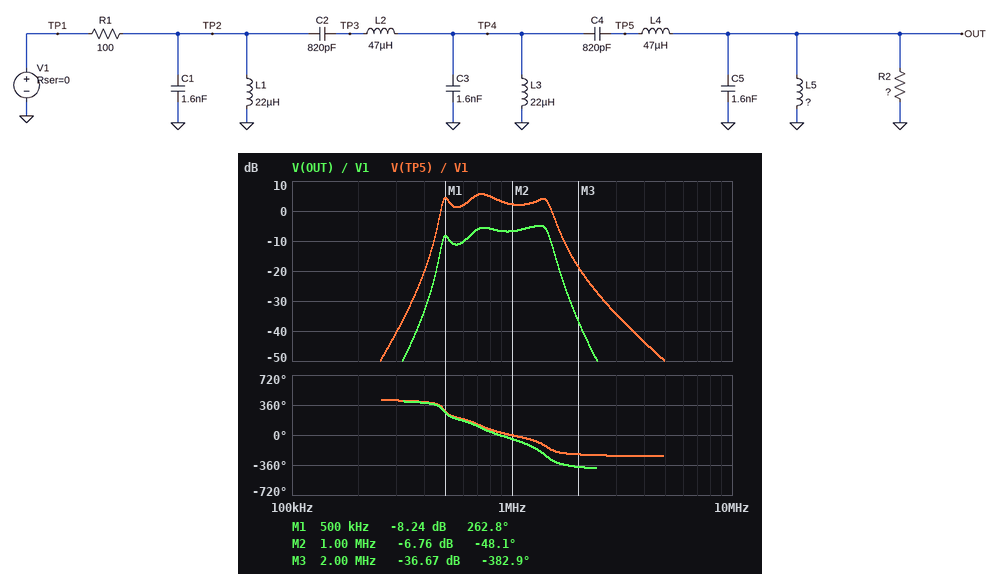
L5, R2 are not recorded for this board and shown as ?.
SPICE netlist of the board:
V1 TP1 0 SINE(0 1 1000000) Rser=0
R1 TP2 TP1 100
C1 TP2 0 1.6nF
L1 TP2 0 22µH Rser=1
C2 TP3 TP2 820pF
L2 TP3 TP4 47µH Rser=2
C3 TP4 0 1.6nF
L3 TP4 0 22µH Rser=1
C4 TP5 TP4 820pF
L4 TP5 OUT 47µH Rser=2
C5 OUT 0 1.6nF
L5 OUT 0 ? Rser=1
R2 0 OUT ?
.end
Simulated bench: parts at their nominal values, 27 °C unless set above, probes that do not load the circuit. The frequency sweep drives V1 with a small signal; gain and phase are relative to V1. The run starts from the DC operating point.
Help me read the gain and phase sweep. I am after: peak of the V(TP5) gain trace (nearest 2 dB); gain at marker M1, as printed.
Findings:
6 dB
-8.24 dB
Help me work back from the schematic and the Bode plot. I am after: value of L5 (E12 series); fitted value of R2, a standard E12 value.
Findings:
12 µH
150 Ω
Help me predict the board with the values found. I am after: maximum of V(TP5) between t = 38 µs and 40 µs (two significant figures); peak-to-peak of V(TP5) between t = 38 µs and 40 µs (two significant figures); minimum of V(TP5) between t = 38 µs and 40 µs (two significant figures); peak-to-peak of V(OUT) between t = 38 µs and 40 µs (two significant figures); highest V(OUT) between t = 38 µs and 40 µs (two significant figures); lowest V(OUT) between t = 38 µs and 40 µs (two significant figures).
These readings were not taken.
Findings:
1.3 V
2.6 V
-1.3 V
920 mV
460 mV
-460 mV
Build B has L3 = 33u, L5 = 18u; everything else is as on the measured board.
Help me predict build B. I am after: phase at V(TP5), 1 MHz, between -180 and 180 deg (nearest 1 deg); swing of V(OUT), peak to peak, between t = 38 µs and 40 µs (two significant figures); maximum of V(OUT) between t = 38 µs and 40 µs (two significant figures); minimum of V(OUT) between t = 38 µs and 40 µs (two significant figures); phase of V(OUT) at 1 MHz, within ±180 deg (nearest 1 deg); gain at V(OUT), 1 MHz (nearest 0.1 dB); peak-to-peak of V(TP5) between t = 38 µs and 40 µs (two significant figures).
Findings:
-7 deg
1.2 V
580 mV
-580 mV
-79 deg
-4.8 dB
2.4 V
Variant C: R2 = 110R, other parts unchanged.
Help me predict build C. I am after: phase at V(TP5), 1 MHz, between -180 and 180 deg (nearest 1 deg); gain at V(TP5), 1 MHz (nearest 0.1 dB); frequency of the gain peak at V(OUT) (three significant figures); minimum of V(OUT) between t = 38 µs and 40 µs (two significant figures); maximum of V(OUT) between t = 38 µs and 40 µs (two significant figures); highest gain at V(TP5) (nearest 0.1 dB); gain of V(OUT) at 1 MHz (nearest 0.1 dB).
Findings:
1 deg
2.4 dB
1.35 MHz
-390 mV
390 mV
5.4 dB
-8.1 dB
